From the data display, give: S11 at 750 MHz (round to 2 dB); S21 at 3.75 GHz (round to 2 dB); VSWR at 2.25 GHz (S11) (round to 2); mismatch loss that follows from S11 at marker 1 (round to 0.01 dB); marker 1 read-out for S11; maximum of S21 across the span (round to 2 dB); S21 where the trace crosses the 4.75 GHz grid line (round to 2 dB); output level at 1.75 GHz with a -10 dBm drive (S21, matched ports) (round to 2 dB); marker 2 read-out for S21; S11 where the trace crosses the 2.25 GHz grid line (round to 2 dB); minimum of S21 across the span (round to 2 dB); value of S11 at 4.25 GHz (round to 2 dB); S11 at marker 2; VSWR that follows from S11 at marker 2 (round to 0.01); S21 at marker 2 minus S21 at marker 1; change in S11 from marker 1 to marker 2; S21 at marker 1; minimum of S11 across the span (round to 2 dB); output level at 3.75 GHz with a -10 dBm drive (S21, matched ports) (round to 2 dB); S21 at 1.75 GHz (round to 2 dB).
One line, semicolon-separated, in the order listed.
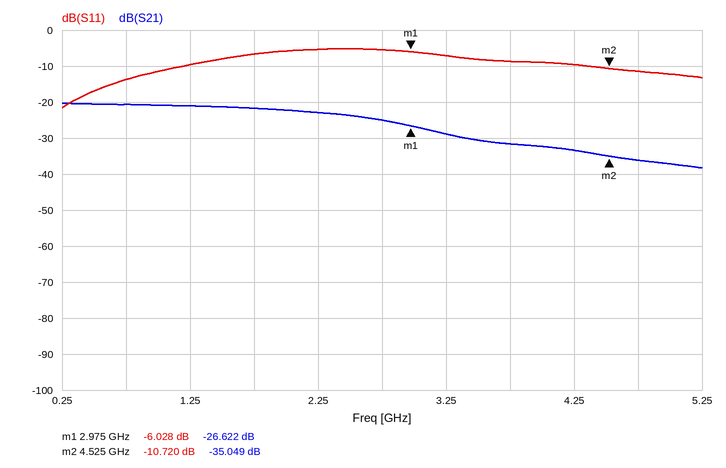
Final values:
-14 dB; -32 dB; 4; 1.25 dB; -6.028 dB; -20 dB; -36 dB; -32 dBm; -35.049 dB; -6 dB; -38 dB; -10 dB; -10.720 dB; 1.82; -8.427 dB; -4.692 dB; -26.622 dB; -22 dB; -42 dBm; -22 dB
